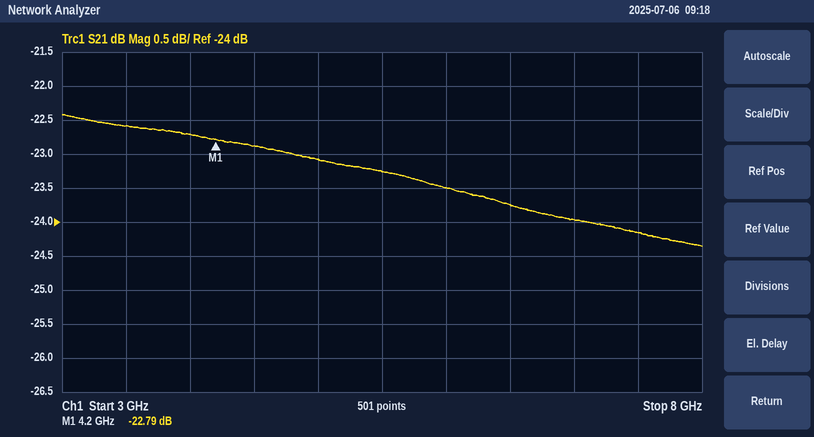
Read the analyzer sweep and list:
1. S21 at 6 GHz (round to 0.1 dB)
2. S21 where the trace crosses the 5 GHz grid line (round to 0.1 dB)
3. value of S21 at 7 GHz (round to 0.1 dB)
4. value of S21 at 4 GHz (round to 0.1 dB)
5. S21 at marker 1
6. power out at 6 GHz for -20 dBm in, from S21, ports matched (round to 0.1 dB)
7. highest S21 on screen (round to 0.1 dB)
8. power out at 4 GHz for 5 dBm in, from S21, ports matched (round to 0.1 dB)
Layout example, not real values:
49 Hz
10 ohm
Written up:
-23.5 dB
-23.1 dB
-24.0 dB
-22.7 dB
-22.79 dB
-43.5 dBm
-22.4 dB
-17.7 dBm
